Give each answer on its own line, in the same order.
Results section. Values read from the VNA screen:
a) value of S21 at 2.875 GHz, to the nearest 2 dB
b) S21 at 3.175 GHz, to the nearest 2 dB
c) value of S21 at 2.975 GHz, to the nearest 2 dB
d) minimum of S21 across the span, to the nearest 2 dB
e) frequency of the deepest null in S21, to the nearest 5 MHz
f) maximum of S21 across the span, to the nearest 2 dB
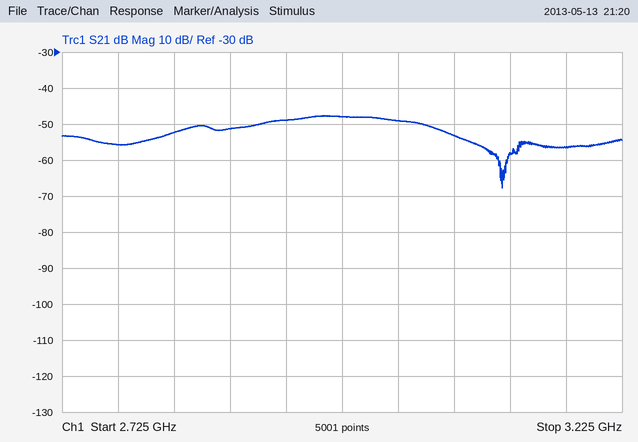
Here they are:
-52 dB
-56 dB
-48 dB
-68 dB
3.120 GHz
-48 dB
